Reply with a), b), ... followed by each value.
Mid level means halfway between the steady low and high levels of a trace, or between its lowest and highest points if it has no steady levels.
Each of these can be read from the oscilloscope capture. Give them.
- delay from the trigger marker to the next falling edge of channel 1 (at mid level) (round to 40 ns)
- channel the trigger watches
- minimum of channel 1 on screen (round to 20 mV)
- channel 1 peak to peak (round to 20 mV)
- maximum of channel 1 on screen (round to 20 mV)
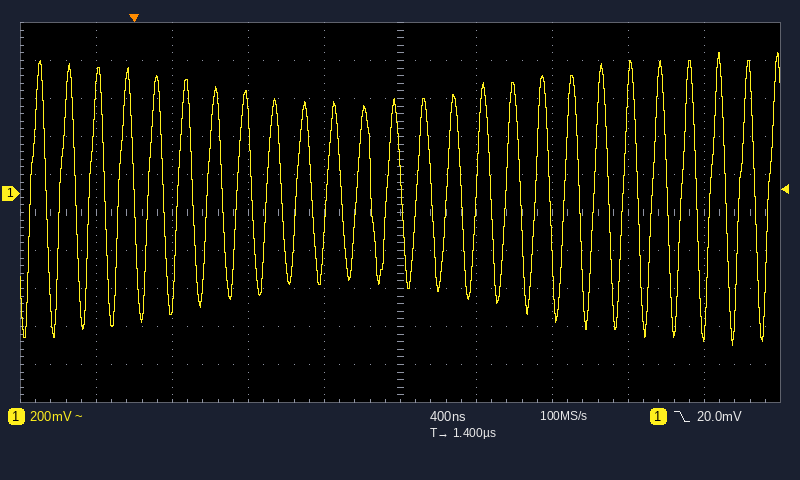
a) 160 ns
b) channel 1
c) -800 mV
d) 1.54 V
e) 740 mV
